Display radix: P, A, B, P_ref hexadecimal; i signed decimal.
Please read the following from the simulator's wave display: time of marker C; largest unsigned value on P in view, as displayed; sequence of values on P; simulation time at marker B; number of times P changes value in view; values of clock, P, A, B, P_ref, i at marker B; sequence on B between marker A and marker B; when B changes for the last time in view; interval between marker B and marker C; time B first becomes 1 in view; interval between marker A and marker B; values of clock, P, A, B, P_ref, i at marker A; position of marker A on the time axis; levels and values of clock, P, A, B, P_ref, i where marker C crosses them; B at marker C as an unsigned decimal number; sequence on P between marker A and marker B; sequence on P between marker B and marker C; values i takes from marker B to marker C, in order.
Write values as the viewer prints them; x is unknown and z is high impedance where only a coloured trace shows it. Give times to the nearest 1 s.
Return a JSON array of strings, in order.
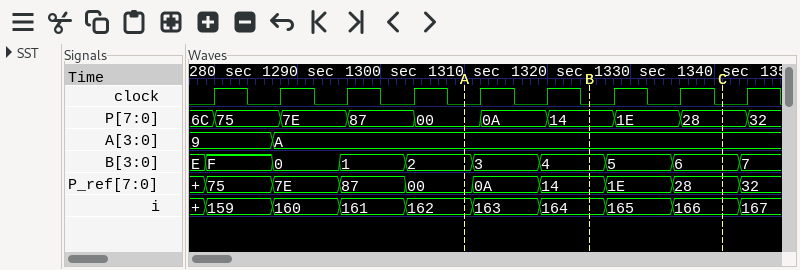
["1341 s", "87", "6C, 75, 7E, 87, 00, 0A, 14, 1E, 28, 32", "1325 s", "9", "clock=0, P=14, A=A, B=4, P_ref=14, i=164", "2, 3, 4", "1343 s", "16 s", "1295 s", "15 s", "clock=0, P=00, A=A, B=2, P_ref=00, i=162", "1310 s", "clock=0, P=28, A=A, B=6, P_ref=28, i=166", "6", "00, 0A, 14", "14, 1E, 28", "164, 165, 166"]
